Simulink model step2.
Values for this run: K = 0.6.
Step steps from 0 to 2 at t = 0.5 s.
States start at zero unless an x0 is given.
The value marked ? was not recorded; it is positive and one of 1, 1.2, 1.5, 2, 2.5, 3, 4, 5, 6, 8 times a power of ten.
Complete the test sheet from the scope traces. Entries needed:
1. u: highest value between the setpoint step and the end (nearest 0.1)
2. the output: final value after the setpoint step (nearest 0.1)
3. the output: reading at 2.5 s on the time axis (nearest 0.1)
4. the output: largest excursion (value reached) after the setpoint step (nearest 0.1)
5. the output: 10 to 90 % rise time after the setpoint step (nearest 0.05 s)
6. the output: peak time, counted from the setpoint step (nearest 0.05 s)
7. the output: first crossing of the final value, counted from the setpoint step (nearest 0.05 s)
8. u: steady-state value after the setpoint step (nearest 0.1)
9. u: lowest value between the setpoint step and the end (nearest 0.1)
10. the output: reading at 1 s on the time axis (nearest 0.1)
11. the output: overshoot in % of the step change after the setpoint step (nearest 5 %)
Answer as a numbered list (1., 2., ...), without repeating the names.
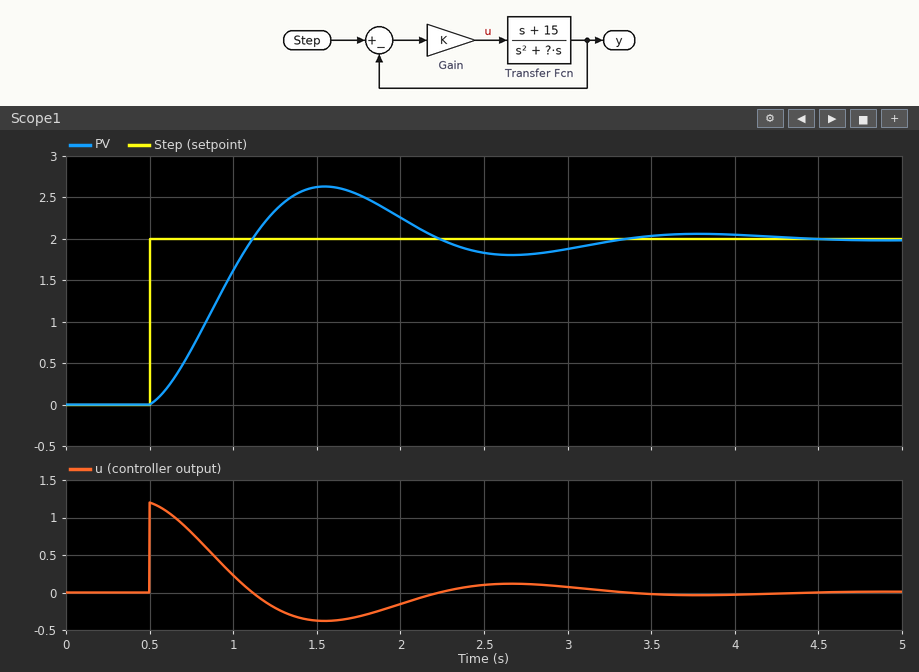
1. 1.2
2. 2.0
3. 1.8
4. 2.6
5. 0.45 s
6. 1.05 s
7. 0.60 s
8. 0.0
9. -0.4
10. 1.6
11. 30 %
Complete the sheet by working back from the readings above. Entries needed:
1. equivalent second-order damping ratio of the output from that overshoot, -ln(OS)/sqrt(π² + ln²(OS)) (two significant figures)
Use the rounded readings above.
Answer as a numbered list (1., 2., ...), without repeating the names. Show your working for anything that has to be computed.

1. ln(0.3) = -1.204; 1.204 / sqrt(9.870 + 1.450) = 0.36
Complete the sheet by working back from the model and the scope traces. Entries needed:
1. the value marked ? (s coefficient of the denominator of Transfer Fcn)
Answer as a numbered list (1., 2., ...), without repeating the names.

1. 1.5
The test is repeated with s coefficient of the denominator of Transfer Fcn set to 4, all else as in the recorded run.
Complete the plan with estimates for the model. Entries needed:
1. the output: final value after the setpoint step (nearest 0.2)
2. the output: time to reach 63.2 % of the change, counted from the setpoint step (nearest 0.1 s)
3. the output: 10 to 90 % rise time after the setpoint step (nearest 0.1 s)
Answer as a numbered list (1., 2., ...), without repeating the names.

1. 2.0
2. 0.5 s
3. 0.8 s
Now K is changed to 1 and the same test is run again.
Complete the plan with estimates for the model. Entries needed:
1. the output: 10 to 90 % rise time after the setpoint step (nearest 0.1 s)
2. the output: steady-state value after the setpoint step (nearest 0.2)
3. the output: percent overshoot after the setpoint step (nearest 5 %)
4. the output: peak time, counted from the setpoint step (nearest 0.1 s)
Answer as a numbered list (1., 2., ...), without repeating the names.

1. 0.3 s
2. 2.0
3. 35 %
4. 0.8 s
